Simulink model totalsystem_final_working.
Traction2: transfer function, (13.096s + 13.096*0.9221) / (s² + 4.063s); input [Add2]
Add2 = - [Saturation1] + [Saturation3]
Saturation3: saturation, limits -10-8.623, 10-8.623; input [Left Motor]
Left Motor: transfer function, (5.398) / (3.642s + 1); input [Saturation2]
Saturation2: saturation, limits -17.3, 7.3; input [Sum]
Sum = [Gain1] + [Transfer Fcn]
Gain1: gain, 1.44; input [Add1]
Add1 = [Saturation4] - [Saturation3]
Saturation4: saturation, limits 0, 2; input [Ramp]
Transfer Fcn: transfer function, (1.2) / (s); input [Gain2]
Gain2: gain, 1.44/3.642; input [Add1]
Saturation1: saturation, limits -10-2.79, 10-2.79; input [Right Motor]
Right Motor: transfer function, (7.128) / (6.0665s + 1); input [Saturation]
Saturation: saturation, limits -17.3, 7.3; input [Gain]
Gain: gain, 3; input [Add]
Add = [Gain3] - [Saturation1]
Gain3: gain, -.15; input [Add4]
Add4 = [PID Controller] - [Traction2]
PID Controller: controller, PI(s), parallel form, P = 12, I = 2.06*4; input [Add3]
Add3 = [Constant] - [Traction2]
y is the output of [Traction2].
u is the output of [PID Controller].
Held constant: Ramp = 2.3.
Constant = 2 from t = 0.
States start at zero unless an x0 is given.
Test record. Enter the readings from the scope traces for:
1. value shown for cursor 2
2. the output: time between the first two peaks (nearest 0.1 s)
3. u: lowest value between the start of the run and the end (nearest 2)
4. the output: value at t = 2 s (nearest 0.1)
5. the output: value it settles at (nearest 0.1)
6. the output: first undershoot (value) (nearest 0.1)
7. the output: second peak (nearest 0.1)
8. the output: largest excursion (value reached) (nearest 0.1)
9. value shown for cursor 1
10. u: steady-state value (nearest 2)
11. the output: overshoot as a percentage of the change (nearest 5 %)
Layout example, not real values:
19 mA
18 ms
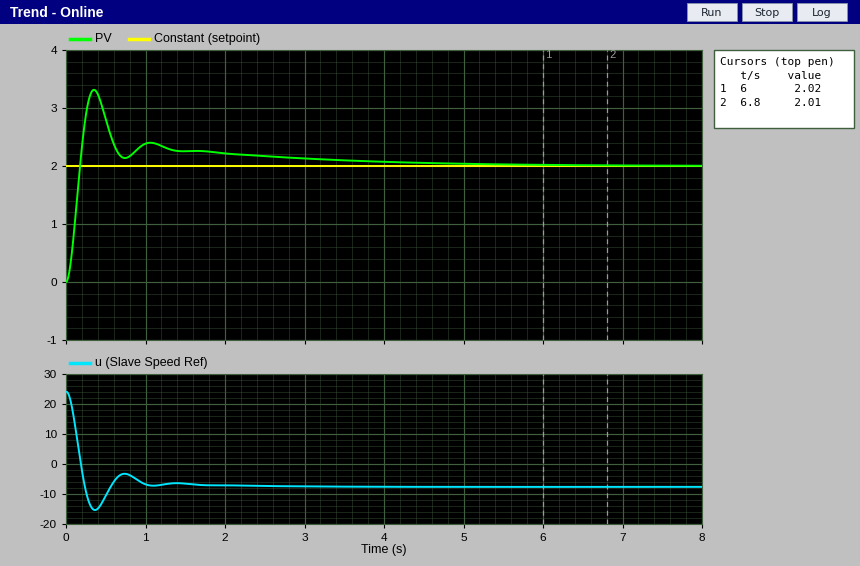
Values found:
2.01
0.7 s
-16
2.2
2.0
2.1
2.4
3.3
2.02
-8
65 %
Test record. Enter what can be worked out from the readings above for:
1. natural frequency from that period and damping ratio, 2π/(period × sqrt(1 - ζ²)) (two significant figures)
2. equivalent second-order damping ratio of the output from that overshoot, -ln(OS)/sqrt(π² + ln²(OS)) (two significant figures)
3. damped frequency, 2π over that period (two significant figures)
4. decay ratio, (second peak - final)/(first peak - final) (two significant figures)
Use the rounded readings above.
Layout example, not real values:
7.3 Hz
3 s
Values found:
9.1 rad/s
0.14
9.0 rad/s
0.31
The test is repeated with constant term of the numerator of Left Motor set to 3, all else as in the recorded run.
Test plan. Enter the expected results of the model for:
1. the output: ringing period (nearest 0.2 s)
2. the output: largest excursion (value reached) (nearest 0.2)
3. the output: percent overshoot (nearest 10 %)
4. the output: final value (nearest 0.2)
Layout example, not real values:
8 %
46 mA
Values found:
0.6 s
3.0
50 %
2.0
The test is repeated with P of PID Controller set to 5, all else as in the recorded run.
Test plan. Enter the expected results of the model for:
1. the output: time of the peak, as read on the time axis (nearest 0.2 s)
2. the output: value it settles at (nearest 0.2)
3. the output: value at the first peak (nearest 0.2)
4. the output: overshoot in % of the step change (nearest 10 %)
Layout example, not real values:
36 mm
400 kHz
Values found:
0.6 s
2.0
3.8
90 %
